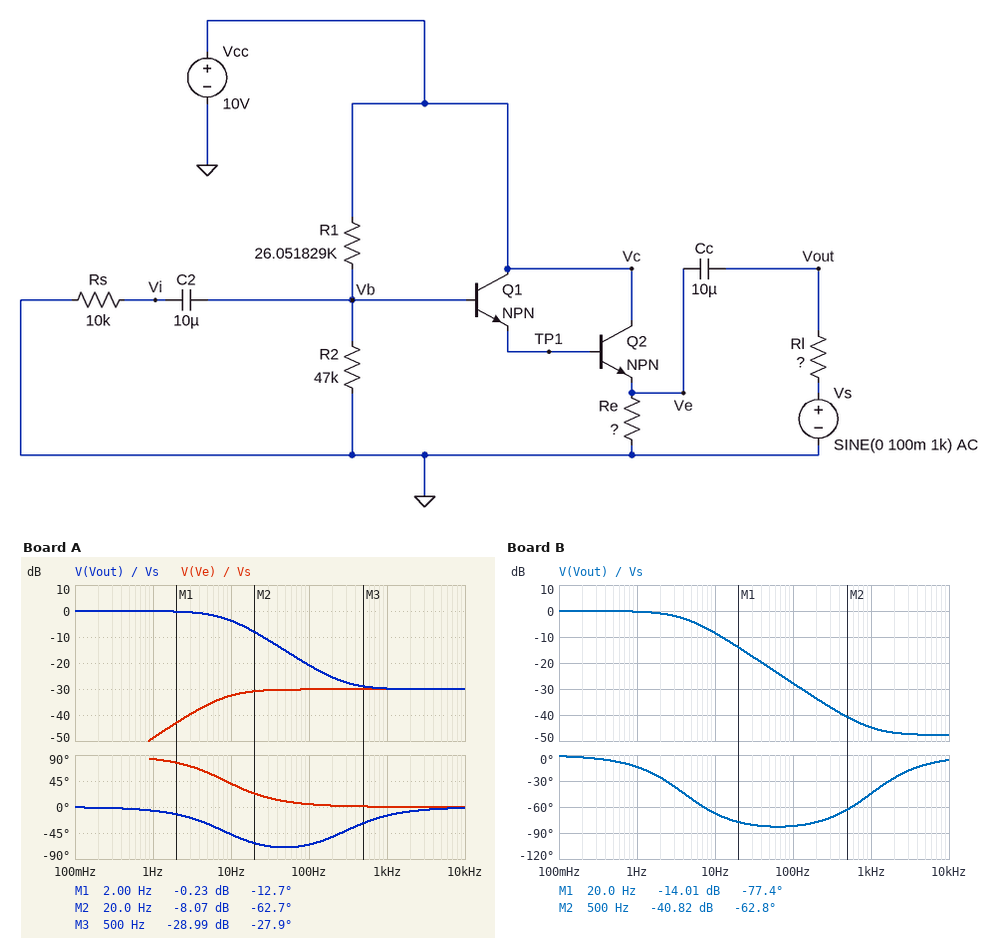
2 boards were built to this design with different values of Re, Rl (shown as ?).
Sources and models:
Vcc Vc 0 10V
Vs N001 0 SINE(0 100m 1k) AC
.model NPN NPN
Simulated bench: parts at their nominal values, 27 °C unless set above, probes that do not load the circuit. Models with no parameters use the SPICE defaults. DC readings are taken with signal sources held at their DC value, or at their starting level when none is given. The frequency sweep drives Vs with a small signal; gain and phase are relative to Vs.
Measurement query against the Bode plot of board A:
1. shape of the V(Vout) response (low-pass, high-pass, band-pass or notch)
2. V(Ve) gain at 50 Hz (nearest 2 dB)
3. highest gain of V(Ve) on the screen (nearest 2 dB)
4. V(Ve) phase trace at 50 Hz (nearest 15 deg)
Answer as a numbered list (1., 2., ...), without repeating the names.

1. low-pass
2. -30 dB
3. -30 dB
4. 15 deg
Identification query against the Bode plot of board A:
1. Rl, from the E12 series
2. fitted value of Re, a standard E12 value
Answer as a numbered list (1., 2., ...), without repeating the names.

1. 1.8 kΩ
2. 5.6 kΩ
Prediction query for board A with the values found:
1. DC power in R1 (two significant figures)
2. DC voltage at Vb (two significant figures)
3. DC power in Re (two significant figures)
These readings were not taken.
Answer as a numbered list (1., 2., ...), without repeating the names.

1. 490 µW
2. 6.4 V
3. 4.5 mW
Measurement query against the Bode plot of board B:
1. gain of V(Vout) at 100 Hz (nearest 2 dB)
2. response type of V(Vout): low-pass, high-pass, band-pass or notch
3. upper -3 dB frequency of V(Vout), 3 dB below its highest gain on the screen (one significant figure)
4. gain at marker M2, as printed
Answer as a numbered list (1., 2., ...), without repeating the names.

1. -28 dB
2. low-pass
3. 4 Hz
4. -40.82 dB
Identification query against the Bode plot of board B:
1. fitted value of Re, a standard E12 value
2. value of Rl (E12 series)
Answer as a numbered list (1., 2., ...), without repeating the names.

1. 1.5 kΩ
2. 3.9 kΩ
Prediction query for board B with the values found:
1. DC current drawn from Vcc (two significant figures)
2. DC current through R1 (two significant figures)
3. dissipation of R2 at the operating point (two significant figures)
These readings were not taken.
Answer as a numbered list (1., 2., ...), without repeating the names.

1. 3.4 mA
2. 140 µA
3. 880 µW
